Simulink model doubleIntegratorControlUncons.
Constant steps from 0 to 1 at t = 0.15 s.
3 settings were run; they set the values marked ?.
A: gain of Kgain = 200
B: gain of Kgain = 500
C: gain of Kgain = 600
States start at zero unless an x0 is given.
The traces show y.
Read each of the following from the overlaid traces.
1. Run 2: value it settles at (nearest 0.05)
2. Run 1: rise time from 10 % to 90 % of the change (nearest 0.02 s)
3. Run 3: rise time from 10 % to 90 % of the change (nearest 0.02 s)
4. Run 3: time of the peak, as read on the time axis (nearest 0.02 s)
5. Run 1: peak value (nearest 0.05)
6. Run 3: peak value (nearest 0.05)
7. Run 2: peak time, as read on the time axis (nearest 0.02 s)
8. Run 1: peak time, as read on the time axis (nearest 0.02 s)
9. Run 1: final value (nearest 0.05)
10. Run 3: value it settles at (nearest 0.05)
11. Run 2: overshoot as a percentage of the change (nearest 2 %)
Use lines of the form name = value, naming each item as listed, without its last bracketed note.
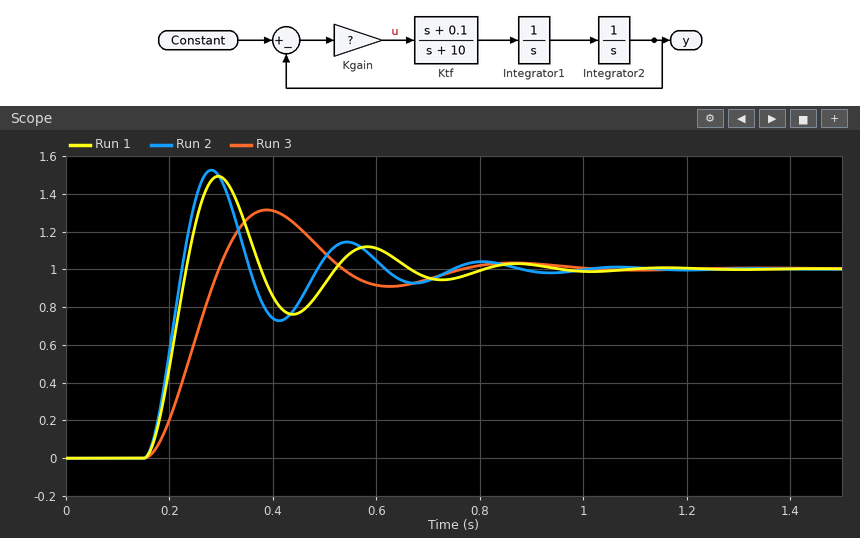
Run 2: value it settles at = 1.00
Run 1: rise time from 10 % to 90 % of the change = 0.06 s
Run 3: rise time from 10 % to 90 % of the change = 0.10 s
Run 3: time of the peak, as read on the time axis = 0.38 s
Run 1: peak value = 1.50
Run 3: peak value = 1.30
Run 2: peak time, as read on the time axis = 0.28 s
Run 1: peak time, as read on the time axis = 0.30 s
Run 1: final value = 1.00
Run 3: value it settles at = 1.00
Run 2: overshoot as a percentage of the change = 52 %
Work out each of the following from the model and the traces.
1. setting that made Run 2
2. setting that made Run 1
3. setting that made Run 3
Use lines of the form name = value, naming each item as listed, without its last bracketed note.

setting that made Run 2 = C
setting that made Run 1 = B
setting that made Run 3 = A
